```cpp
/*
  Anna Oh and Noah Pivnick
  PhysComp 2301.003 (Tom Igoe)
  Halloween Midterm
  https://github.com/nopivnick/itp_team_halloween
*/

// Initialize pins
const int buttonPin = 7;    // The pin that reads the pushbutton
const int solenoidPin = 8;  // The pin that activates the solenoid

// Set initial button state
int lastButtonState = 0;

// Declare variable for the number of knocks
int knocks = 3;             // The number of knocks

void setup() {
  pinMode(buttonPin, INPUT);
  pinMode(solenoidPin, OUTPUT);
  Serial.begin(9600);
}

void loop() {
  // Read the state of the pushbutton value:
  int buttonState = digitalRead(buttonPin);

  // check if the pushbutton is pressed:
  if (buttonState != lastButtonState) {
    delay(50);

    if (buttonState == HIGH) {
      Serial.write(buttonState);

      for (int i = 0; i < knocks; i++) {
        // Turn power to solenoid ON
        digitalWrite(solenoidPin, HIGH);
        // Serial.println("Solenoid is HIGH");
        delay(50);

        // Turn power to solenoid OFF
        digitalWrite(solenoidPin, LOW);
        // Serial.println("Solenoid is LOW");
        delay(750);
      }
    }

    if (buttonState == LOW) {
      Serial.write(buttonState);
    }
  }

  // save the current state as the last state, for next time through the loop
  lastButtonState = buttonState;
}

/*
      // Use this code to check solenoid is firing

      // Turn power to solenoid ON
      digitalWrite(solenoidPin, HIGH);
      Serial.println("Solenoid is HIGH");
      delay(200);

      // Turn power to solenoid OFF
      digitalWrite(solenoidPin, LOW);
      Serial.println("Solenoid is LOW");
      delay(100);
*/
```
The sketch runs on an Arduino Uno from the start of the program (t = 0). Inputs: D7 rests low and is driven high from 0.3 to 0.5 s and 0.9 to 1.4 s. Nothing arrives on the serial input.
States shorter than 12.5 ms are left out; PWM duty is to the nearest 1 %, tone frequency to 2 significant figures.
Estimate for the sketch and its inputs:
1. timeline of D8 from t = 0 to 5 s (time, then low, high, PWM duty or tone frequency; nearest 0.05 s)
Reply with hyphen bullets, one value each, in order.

- 0 s low; 0.35 s high; 0.4 s low; 1.15 s high; 1.2 s low; 1.95 s high; 2 s low
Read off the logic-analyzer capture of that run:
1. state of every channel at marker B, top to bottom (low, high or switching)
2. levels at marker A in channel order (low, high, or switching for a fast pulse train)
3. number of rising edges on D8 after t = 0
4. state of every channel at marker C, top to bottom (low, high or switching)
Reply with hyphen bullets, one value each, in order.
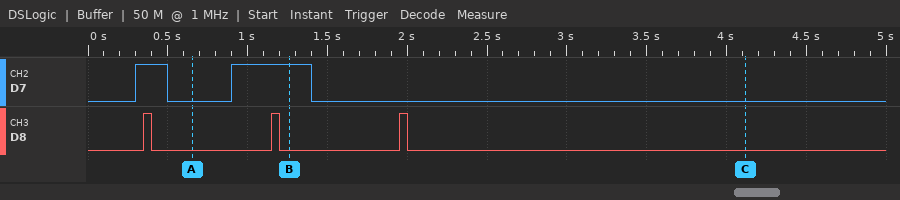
- D7 high, D8 low
- D7 low, D8 low
- 3
- D7 low, D8 low
